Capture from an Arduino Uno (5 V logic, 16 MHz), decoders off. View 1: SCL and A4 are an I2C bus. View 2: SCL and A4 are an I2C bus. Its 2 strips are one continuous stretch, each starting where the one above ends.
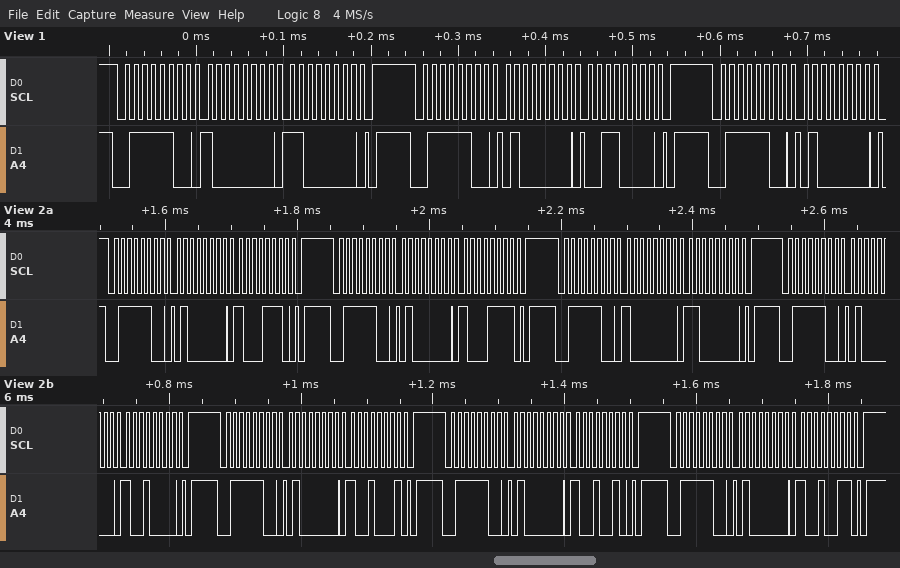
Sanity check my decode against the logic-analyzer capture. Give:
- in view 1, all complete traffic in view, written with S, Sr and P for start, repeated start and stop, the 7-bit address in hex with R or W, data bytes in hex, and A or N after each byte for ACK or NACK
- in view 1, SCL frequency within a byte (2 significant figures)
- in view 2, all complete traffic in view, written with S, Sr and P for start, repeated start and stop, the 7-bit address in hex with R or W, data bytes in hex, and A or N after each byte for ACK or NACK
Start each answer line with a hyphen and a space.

- S 3EW A 80 A C0 A P S 3EW A 40 A 30 A P S 3EW A 40 A
- 100 kHz
- S 3EW A 40 A 8E A P S 3EW A 40 A 8F A P S 3EW A 80 A C0 A P S 3EW A 40 A 90 A P S 3EW A 40 A 91 A P S 3EW A 40 A 92 A P S 3EW A 40 A 93 A P
